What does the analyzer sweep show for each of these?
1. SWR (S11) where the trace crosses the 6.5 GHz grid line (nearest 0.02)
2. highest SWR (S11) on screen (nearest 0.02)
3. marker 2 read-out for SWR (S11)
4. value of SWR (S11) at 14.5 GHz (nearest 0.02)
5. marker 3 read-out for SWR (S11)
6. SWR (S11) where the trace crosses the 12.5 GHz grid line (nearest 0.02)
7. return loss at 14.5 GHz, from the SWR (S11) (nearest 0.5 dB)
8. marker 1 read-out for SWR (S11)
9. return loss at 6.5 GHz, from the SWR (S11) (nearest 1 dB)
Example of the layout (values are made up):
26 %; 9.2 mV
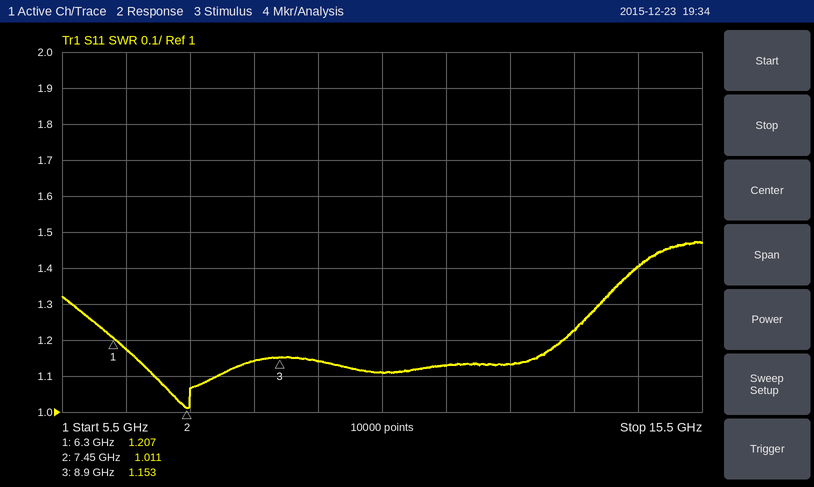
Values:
1.18; 1.48; 1.011; 1.40; 1.153; 1.14; 15.5 dB; 1.207; 22 dB
